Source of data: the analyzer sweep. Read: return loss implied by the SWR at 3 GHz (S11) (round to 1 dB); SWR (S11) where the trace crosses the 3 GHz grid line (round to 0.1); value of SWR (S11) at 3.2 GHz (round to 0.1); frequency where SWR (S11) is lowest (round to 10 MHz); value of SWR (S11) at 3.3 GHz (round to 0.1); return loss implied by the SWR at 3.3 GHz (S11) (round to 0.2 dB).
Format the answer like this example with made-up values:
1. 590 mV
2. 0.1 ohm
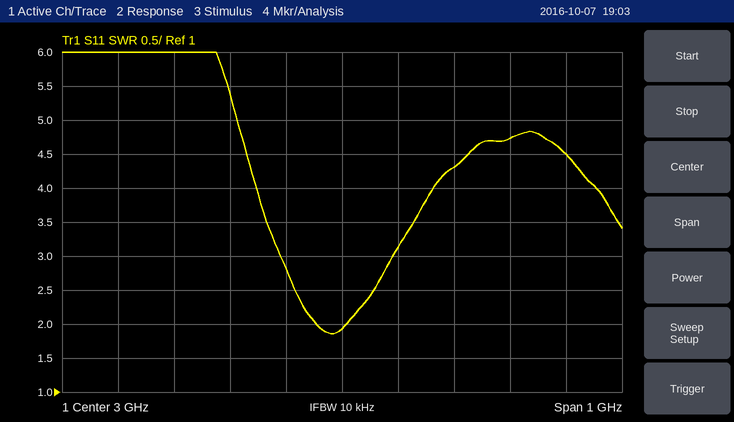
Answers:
1. 10 dB
2. 1.9
3. 4.3
4. 2.98 GHz
5. 4.7
6. 3.8 dB
